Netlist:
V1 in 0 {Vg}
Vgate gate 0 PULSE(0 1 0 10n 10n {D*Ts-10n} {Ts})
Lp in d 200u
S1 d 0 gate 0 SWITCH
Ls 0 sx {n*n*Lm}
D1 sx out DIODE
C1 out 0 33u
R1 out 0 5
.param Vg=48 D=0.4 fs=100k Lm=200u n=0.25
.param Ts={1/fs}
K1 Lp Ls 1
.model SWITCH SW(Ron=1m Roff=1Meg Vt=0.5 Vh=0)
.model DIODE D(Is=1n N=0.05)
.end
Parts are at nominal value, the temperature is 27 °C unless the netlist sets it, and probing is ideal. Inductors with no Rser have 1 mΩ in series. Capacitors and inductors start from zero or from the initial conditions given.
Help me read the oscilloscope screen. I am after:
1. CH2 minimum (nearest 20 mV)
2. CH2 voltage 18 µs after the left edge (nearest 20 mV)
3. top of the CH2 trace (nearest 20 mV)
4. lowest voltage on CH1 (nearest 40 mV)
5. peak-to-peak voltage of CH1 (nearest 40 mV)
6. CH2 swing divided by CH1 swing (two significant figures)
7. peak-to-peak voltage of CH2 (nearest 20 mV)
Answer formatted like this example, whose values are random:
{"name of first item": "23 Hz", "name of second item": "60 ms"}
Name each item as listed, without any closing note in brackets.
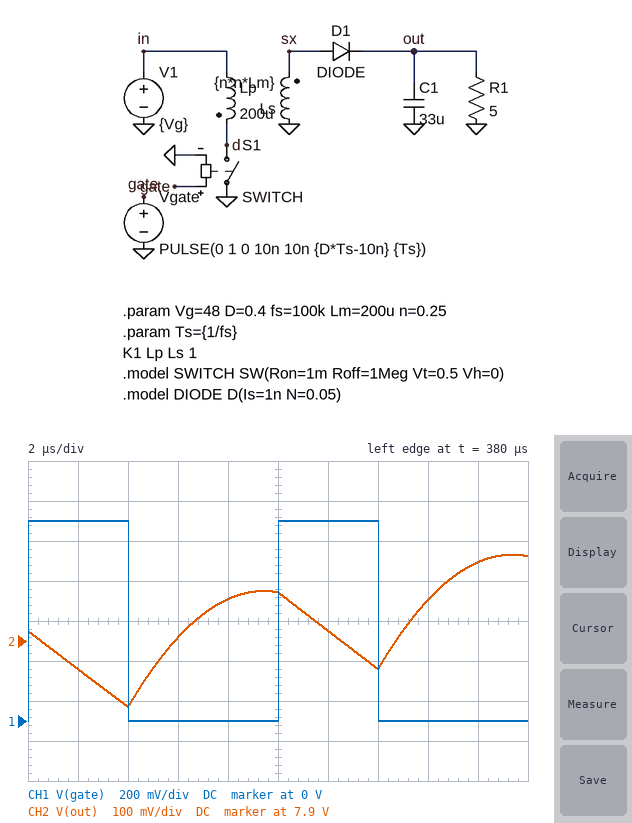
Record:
{"CH2 minimum": "7.74 V", "CH2 voltage 18 µs after the left edge": "8.10 V", "top of the CH2 trace": "8.12 V", "lowest voltage on CH1": "0 V", "peak-to-peak voltage of CH1": "1.00 V", "CH2 swing divided by CH1 swing": "0.38", "peak-to-peak voltage of CH2": "380 mV"}
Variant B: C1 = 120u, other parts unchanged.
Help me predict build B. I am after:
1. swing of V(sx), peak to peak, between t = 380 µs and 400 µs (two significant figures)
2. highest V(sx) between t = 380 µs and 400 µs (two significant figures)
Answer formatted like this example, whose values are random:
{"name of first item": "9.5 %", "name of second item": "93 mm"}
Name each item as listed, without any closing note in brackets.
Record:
{"swing of V(sx), peak to peak, between t = 380 µs and 400 µs": "24 V", "highest V(sx) between t = 380 µs and 400 µs": "12 V"}
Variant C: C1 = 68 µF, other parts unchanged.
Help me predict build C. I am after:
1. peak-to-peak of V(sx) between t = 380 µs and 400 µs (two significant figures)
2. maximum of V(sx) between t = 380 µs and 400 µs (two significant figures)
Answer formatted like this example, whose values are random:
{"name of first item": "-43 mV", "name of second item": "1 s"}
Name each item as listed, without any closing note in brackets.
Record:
{"peak-to-peak of V(sx) between t = 380 µs and 400 µs": "21 V", "maximum of V(sx) between t = 380 µs and 400 µs": "9.4 V"}
